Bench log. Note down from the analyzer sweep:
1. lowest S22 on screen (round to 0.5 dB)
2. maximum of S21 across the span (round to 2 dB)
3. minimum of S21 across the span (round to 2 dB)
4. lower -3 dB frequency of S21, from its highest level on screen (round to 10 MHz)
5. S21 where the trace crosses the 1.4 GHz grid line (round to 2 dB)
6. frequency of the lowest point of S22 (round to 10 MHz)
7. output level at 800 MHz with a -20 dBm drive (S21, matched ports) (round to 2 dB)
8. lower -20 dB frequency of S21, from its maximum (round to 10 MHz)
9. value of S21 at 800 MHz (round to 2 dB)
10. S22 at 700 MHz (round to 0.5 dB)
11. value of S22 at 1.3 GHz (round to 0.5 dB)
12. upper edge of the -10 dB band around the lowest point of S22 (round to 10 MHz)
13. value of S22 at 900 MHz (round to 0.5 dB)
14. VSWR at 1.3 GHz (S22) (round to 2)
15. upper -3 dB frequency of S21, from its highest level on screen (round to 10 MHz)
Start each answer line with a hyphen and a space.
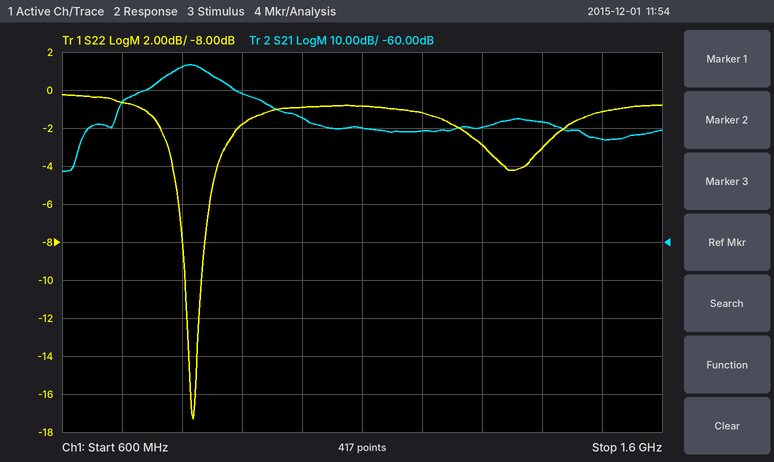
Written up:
- -17.5 dB
- -14 dB
- -42 dB
- 770 MHz
- -28 dB
- 820 MHz
- -34 dBm
- 630 MHz
- -14 dB
- -0.5 dB
- -3.0 dB
- 830 MHz
- -2.0 dB
- 6
- 850 MHz
